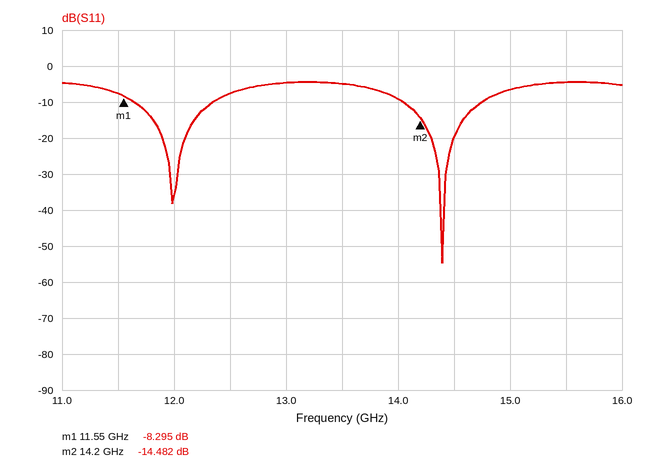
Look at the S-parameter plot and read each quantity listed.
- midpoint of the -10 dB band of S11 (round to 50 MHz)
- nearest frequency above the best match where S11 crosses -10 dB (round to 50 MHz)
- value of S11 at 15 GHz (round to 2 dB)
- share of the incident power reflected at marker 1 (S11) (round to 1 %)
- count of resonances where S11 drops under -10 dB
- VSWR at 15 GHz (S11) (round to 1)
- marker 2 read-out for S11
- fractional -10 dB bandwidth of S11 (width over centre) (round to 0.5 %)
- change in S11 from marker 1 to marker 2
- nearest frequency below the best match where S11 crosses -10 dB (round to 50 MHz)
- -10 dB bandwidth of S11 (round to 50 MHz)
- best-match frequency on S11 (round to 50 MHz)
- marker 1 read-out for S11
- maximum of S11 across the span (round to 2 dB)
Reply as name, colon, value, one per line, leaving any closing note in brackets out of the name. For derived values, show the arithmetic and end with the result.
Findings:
midpoint of the -10 dB band of S11: 14.40 GHz
nearest frequency above the best match where S11 crosses -10 dB: 14.75 GHz
value of S11 at 15 GHz: -6 dB
share of the incident power reflected at marker 1 (S11): 10^(-8.295/10) ≈ 15 %
count of resonances where S11 drops under -10 dB: 2
VSWR at 15 GHz (S11): |Γ| = 10^(-6/20) = 0.5012; VSWR = (1 + 0.5012)/(1 − 0.5012) ≈ 3
marker 2 read-out for S11: -14.482 dB
fractional -10 dB bandwidth of S11 (width over centre): 700 MHz / 14.4 GHz ≈ 4.86 %, so 5.0 % to the nearest 0.5 %
change in S11 from marker 1 to marker 2: -14.482 − (-8.295) = -6.187 dB
nearest frequency below the best match where S11 crosses -10 dB: 14.05 GHz
-10 dB bandwidth of S11: 14.75 GHz − 14.05 GHz = 700 MHz
best-match frequency on S11: 14.40 GHz
marker 1 read-out for S11: -8.295 dB
maximum of S11 across the span: -4 dB
